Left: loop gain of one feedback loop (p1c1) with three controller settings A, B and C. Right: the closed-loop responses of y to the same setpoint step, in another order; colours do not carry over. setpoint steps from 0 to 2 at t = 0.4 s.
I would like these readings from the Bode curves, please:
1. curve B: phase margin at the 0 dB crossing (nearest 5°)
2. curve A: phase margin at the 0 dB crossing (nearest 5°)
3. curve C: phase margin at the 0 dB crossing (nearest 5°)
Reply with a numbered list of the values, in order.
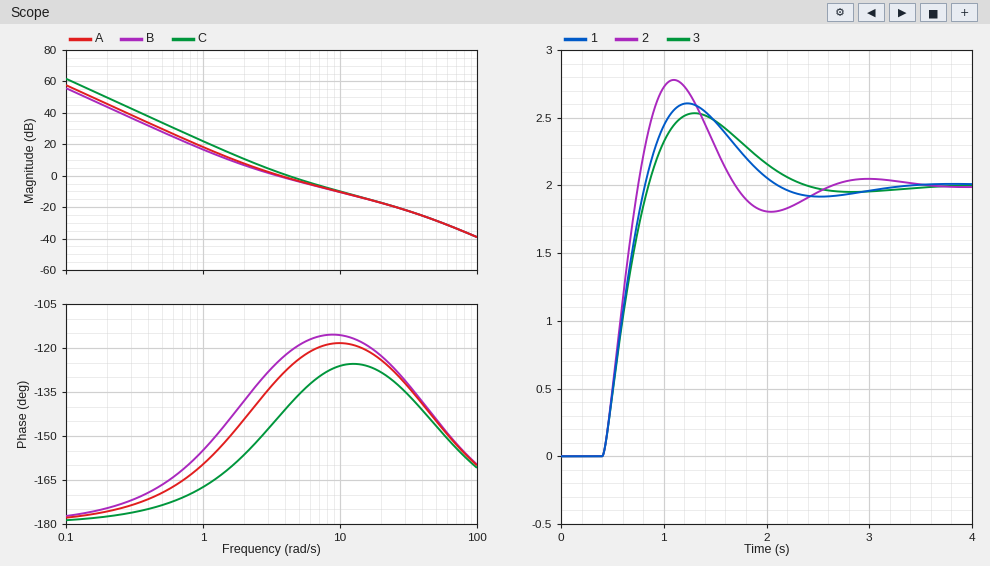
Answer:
1. 55°
2. 50°
3. 40°
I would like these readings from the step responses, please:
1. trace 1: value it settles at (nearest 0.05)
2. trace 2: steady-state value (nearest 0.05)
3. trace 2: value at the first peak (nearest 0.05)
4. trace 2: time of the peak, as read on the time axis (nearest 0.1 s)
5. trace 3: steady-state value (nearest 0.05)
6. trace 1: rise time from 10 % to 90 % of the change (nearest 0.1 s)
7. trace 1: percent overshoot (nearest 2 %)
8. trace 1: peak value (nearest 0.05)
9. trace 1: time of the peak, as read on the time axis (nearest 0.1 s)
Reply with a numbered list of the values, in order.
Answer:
1. 2.00
2. 2.00
3. 2.80
4. 1.1 s
5. 2.00
6. 0.3 s
7. 30 %
8. 2.60
9. 1.2 s
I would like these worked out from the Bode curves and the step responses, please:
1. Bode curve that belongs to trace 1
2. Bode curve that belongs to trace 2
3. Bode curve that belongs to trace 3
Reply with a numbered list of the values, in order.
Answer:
1. A
2. C
3. B
